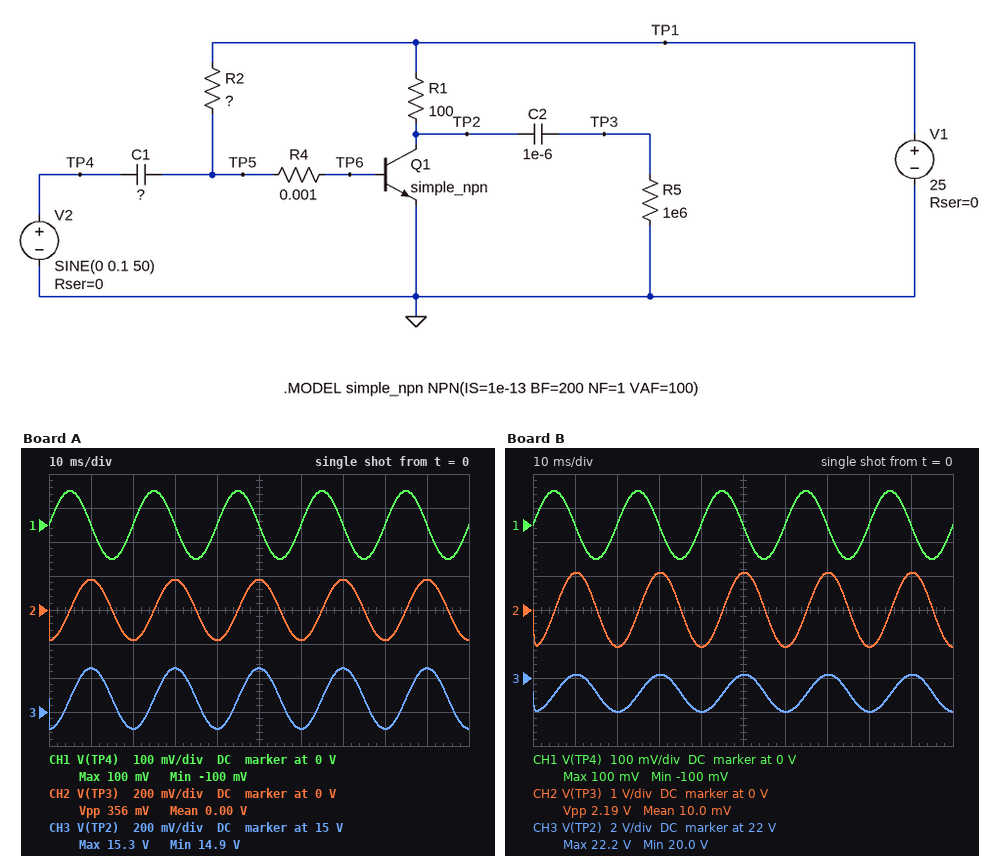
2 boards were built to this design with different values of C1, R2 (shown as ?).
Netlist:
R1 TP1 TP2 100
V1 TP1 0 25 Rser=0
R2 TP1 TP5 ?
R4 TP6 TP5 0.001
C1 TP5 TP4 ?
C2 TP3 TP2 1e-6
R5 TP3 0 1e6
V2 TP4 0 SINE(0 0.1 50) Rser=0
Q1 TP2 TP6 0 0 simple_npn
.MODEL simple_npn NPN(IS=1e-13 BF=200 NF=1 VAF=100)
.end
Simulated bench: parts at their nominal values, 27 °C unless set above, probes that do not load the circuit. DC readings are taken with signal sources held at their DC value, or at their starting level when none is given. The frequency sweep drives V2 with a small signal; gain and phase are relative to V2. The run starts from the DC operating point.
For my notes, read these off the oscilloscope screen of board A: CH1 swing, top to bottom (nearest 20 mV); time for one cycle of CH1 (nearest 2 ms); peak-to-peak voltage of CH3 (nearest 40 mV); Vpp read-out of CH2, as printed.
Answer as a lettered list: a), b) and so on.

a) 200 mV
b) 20 ms
c) 360 mV
d) 356 mV
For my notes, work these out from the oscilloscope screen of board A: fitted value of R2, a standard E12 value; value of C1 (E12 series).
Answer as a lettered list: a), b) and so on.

a) 56 kΩ
b) 270 nF
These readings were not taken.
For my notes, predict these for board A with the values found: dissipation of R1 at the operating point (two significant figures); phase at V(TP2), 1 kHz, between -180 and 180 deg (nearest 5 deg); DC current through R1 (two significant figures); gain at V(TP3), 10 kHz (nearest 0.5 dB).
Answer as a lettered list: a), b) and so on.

a) 980 mW
b) -95 deg
c) 99 mA
d) 48.0 dB
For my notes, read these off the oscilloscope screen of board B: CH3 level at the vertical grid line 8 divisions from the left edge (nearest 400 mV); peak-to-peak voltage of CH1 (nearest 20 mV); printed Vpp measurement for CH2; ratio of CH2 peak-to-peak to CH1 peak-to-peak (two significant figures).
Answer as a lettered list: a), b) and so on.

a) 20.0 V
b) 200 mV
c) 2.19 V
d) 11
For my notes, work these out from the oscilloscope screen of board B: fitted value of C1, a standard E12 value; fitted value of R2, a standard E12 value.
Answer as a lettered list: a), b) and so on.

a) 1.5 µF
b) 150 kΩ
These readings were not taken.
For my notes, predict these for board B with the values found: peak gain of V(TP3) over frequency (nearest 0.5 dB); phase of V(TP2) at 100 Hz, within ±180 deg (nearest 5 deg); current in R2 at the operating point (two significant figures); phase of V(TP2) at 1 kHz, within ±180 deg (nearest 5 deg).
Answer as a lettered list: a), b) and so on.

a) 43.5 dB
b) -100 deg
c) 160 µA
d) -145 deg
